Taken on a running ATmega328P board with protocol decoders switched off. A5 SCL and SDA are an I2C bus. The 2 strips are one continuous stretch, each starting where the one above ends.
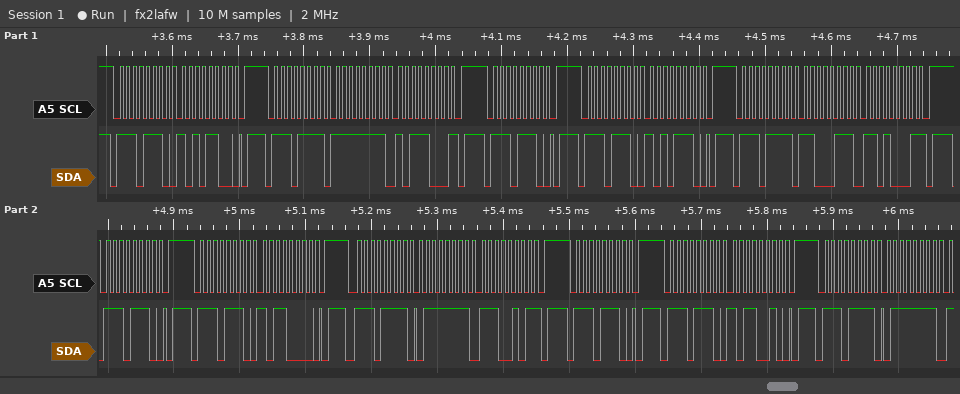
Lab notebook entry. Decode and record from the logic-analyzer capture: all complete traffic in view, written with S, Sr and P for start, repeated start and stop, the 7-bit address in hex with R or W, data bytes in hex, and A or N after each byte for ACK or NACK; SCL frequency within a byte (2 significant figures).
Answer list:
S 77W A AC A P S 77R A FF A B8 N P S 77W A P S 77W A AE A P S 77R A C7 A D1 N P S 77W A P S 77W A B0 A P S 77R A 7F A E5 N P S 77W A P S 77W A B2 A P S 77R A 7F A
100 kHz
